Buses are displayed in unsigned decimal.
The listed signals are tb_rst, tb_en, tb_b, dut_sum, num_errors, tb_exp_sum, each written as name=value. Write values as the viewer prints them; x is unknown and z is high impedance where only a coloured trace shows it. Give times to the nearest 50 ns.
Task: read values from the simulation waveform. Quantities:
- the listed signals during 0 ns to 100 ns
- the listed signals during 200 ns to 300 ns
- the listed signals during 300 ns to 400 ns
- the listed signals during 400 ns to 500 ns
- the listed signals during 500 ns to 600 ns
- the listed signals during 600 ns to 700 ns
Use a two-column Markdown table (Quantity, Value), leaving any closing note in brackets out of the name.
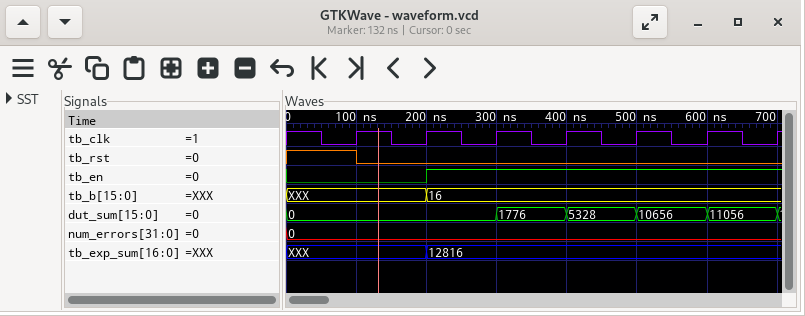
| Quantity | Value |
|---|---|
| the listed signals during 0 ns to 100 ns | tb_rst=1, tb_en=0, tb_b=XXX, dut_sum=0, num_errors=0, tb_exp_sum=XXX |
| the listed signals during 200 ns to 300 ns | tb_rst=0, tb_en=1, tb_b=16, dut_sum=0, num_errors=0, tb_exp_sum=12816 |
| the listed signals during 300 ns to 400 ns | tb_rst=0, tb_en=1, tb_b=16, dut_sum=1776, num_errors=0, tb_exp_sum=12816 |
| the listed signals during 400 ns to 500 ns | tb_rst=0, tb_en=1, tb_b=16, dut_sum=5328, num_errors=0, tb_exp_sum=12816 |
| the listed signals during 500 ns to 600 ns | tb_rst=0, tb_en=1, tb_b=16, dut_sum=10656, num_errors=0, tb_exp_sum=12816 |
| the listed signals during 600 ns to 700 ns | tb_rst=0, tb_en=1, tb_b=16, dut_sum=11056, num_errors=0, tb_exp_sum=12816 |
